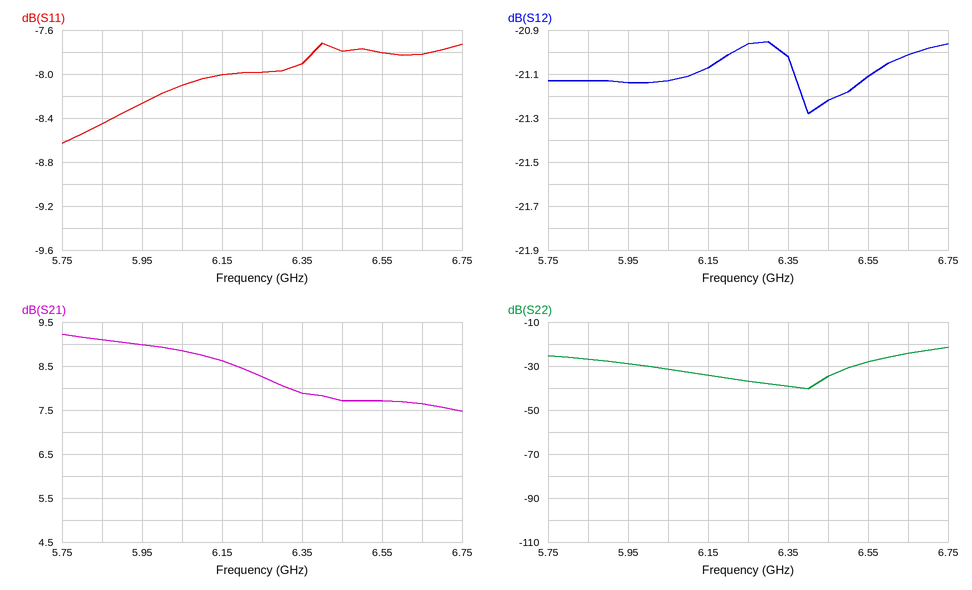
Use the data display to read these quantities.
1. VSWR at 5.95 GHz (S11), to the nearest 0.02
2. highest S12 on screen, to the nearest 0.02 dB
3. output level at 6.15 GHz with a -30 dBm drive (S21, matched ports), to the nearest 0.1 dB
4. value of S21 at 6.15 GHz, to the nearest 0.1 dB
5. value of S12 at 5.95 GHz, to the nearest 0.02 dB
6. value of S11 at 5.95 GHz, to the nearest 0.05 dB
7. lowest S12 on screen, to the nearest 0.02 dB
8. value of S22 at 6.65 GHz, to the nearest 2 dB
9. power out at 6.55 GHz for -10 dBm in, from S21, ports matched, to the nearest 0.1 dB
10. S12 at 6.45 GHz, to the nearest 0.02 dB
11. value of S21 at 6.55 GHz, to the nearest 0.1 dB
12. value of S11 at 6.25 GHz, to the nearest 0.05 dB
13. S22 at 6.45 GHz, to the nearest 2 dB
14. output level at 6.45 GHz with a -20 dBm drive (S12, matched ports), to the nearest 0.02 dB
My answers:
2.26
-20.96 dB
-21.4 dBm
8.6 dB
-21.14 dB
-8.25 dB
-21.28 dB
-24 dB
-2.3 dBm
-21.22 dB
7.7 dB
-8.00 dB
-34 dB
-41.22 dBm
